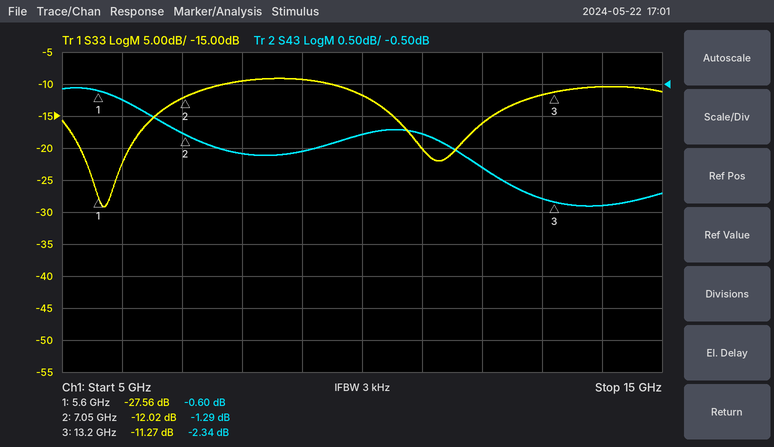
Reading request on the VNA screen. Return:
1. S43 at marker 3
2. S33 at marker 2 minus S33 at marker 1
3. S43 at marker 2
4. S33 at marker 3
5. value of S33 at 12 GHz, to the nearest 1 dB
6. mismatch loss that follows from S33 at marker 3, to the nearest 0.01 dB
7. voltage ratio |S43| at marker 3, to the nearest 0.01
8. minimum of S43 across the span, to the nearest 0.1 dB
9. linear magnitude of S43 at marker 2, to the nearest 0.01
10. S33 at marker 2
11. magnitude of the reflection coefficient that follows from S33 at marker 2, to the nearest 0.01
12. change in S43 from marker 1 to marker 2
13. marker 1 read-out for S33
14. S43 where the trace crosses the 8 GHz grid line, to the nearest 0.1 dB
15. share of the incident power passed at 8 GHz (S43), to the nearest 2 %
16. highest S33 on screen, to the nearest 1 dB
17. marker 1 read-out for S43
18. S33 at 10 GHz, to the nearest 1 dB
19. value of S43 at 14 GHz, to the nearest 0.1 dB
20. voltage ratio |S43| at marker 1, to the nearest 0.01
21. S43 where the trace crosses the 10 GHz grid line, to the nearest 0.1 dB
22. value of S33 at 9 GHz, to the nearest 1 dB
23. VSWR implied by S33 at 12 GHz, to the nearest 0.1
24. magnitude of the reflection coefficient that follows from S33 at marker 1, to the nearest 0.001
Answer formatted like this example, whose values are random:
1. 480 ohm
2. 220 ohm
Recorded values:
1. -2.34 dB
2. 15.54 dB
3. -1.29 dB
4. -11.27 dB
5. -16 dB
6. 0.34 dB
7. 0.76
8. -2.4 dB
9. 0.86
10. -12.02 dB
11. 0.25
12. -0.69 dB
13. -27.56 dB
14. -1.6 dB
15. 70 %
16. -9 dB
17. -0.60 dB
18. -12 dB
19. -2.4 dB
20. 0.93
21. -1.3 dB
22. -9 dB
23. 1.4
24. 0.042
